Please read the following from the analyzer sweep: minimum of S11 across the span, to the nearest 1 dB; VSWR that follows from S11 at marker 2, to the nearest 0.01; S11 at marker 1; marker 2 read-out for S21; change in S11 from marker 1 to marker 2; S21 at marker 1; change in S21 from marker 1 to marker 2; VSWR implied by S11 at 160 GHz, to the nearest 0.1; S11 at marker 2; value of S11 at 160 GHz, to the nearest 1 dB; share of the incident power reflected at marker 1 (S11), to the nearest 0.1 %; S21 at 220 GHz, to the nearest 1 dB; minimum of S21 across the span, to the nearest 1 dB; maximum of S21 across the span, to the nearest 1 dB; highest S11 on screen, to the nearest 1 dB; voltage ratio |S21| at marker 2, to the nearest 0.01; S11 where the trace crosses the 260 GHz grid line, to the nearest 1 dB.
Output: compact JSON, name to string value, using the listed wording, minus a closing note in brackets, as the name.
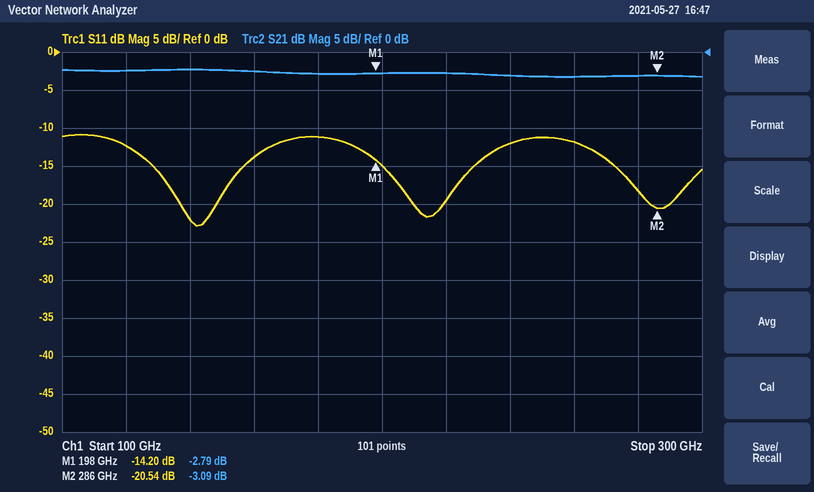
{"minimum of S11 across the span, to the nearest 1 dB": "-23 dB", "VSWR that follows from S11 at marker 2, to the nearest 0.01": "1.21", "S11 at marker 1": "-14.20 dB", "marker 2 read-out for S21": "-3.09 dB", "change in S11 from marker 1 to marker 2": "-6.34 dB", "S21 at marker 1": "-2.79 dB", "change in S21 from marker 1 to marker 2": "-0.30 dB", "VSWR implied by S11 at 160 GHz, to the nearest 0.1": "1.5", "S11 at marker 2": "-20.54 dB", "value of S11 at 160 GHz, to the nearest 1 dB": "-14 dB", "share of the incident power reflected at marker 1 (S11), to the nearest 0.1 %": "3.8 %", "S21 at 220 GHz, to the nearest 1 dB": "-3 dB", "minimum of S21 across the span, to the nearest 1 dB": "-3 dB", "maximum of S21 across the span, to the nearest 1 dB": "-2 dB", "highest S11 on screen, to the nearest 1 dB": "-11 dB", "voltage ratio |S21| at marker 2, to the nearest 0.01": "0.70", "S11 where the trace crosses the 260 GHz grid line, to the nearest 1 dB": "-12 dB"}
